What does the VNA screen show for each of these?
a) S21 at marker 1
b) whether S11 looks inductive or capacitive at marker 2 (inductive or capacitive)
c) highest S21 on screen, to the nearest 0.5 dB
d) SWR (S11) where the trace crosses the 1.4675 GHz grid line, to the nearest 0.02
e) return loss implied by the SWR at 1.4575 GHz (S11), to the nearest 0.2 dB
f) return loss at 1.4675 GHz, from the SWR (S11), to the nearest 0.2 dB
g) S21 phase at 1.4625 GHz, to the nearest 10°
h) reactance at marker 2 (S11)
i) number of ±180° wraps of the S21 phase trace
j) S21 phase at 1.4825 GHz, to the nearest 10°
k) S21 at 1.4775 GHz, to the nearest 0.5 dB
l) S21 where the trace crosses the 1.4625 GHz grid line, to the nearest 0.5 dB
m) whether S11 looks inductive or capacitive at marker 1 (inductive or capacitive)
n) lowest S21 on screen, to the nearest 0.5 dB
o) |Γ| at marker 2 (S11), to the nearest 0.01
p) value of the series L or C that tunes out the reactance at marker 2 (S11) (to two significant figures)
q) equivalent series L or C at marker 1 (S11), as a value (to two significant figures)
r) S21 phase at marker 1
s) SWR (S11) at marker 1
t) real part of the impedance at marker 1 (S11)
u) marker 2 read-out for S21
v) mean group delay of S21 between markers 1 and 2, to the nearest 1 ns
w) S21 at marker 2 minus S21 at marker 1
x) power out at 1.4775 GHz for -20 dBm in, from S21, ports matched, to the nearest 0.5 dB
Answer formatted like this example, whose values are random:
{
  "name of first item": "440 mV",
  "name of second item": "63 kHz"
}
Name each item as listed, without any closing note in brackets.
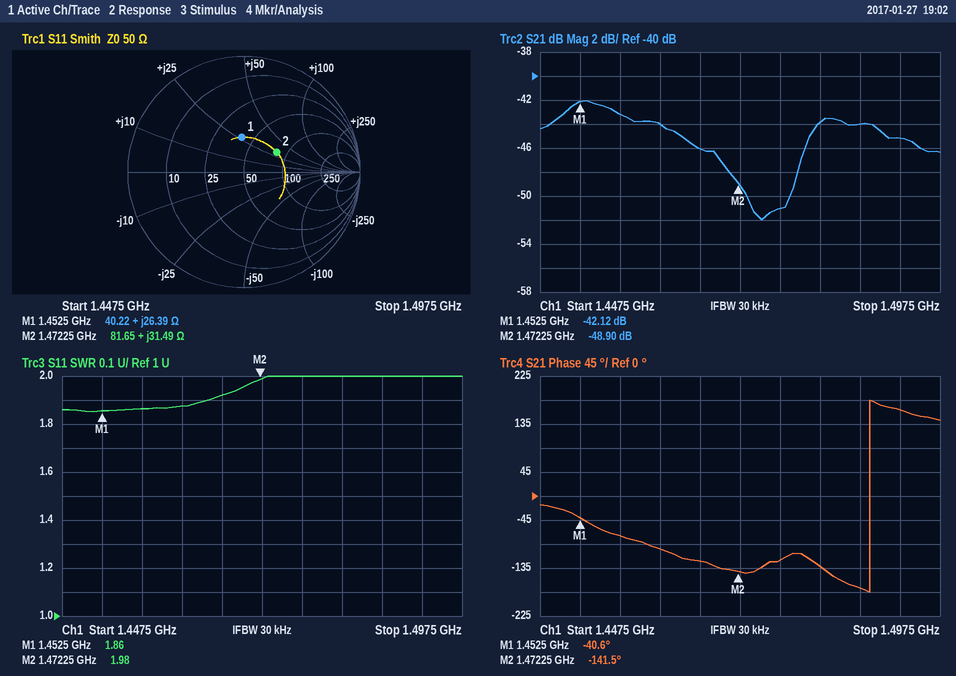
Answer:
{
  "S21 at marker 1": "-42.12 dB",
  "whether S11 looks inductive or capacitive at marker 2": "inductive",
  "highest S21 on screen, to the nearest 0.5 dB": "-42.0 dB",
  "SWR (S11) where the trace crosses the 1.4675 GHz grid line, to the nearest 0.02": "1.92",
  "return loss implied by the SWR at 1.4575 GHz (S11), to the nearest 0.2 dB": "10.4 dB",
  "return loss at 1.4675 GHz, from the SWR (S11), to the nearest 0.2 dB": "10.0 dB",
  "S21 phase at 1.4625 GHz, to the nearest 10°": "-100°",
  "reactance at marker 2": "+31.49 Ω",
  "number of ±180° wraps of the S21 phase trace": "1",
  "S21 phase at 1.4825 GHz, to the nearest 10°": "-130°",
  "S21 at 1.4775 GHz, to the nearest 0.5 dB": "-51.0 dB",
  "S21 where the trace crosses the 1.4625 GHz grid line, to the nearest 0.5 dB": "-44.0 dB",
  "whether S11 looks inductive or capacitive at marker 1": "inductive",
  "lowest S21 on screen, to the nearest 0.5 dB": "-52.0 dB",
  "|Γ| at marker 2 (S11), to the nearest 0.01": "0.33",
  "value of the series L or C that tunes out the reactance at marker 2 (S11)": "3.4 pF",
  "equivalent series L or C at marker 1 (S11), as a value": "2.9 nH",
  "S21 phase at marker 1": "-40.6°",
  "SWR (S11) at marker 1": "1.86",
  "real part of the impedance at marker 1": "40.22 Ω",
  "marker 2 read-out for S21": "-48.90 dB",
  "mean group delay of S21 between markers 1 and 2, to the nearest 1 ns": "14 ns",
  "S21 at marker 2 minus S21 at marker 1": "-6.78 dB",
  "power out at 1.4775 GHz for -20 dBm in, from S21, ports matched, to the nearest 0.5 dB": "-71.0 dBm"
}
